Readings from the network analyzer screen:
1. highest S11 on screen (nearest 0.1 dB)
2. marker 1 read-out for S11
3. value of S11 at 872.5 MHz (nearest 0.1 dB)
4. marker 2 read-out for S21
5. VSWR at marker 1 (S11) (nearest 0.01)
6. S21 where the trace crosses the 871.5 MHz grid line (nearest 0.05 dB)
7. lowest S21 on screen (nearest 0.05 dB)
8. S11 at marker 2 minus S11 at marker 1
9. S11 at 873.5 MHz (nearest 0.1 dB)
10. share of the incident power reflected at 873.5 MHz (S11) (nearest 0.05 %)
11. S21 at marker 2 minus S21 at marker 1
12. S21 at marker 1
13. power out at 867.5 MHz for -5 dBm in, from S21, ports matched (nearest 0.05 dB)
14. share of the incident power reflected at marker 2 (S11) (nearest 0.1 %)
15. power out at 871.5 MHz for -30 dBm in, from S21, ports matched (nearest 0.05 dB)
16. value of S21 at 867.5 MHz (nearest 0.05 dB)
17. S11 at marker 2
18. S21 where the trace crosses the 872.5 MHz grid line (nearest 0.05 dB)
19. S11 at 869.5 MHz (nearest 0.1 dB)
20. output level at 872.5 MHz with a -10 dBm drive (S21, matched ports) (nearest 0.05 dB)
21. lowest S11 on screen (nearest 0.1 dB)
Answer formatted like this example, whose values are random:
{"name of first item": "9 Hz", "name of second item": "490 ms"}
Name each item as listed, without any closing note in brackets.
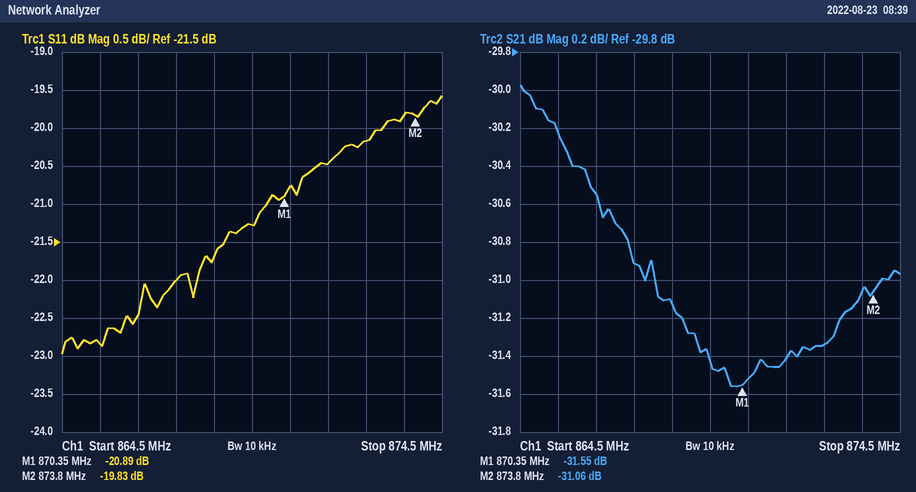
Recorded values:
{"highest S11 on screen": "-19.6 dB", "marker 1 read-out for S11": "-20.89 dB", "value of S11 at 872.5 MHz": "-20.2 dB", "marker 2 read-out for S21": "-31.06 dB", "VSWR at marker 1 (S11)": "1.20", "S21 where the trace crosses the 871.5 MHz grid line": "-31.40 dB", "lowest S21 on screen": "-31.55 dB", "S11 at marker 2 minus S11 at marker 1": "1.06 dB", "S11 at 873.5 MHz": "-19.8 dB", "share of the incident power reflected at 873.5 MHz (S11)": "1.05 %", "S21 at marker 2 minus S21 at marker 1": "0.49 dB", "S21 at marker 1": "-31.55 dB", "power out at 867.5 MHz for -5 dBm in, from S21, ports matched": "-35.90 dBm", "share of the incident power reflected at marker 2 (S11)": "1.0 %", "power out at 871.5 MHz for -30 dBm in, from S21, ports matched": "-61.40 dBm", "value of S21 at 867.5 MHz": "-30.90 dB", "S11 at marker 2": "-19.83 dB", "S21 where the trace crosses the 872.5 MHz grid line": "-31.35 dB", "S11 at 869.5 MHz": "-21.3 dB", "output level at 872.5 MHz with a -10 dBm drive (S21, matched ports)": "-41.35 dBm", "lowest S11 on screen": "-23.0 dB"}
